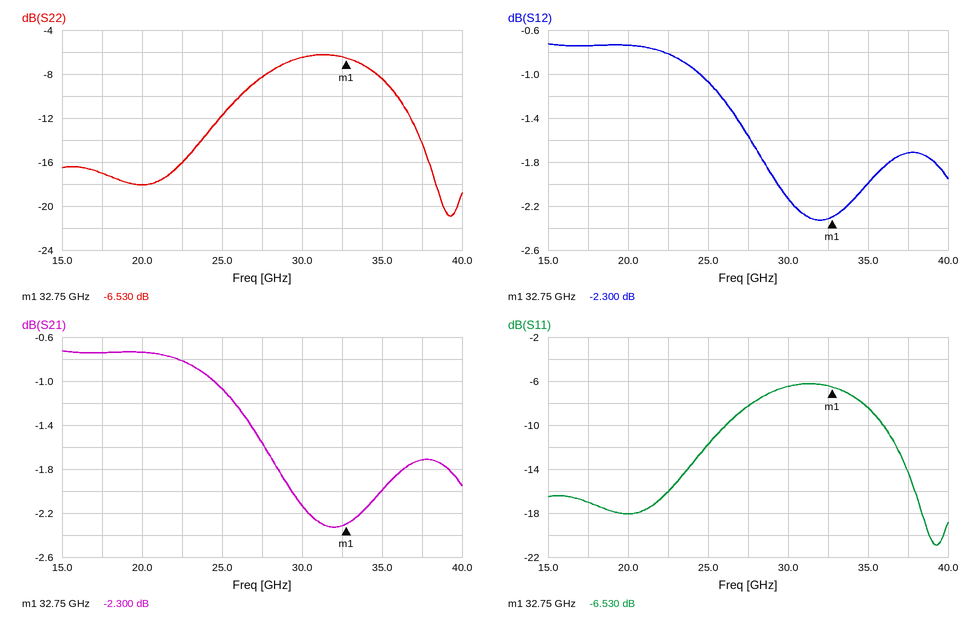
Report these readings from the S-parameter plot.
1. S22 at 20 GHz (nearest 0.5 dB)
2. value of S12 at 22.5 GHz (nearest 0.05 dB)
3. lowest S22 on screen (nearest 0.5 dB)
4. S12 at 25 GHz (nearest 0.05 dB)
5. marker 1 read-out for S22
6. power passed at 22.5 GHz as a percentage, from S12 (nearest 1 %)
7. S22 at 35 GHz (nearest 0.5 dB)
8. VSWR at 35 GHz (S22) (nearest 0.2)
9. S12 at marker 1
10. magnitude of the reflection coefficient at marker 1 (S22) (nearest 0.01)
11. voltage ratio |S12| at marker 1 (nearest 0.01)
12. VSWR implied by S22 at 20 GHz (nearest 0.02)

-18.0 dB
-0.80 dB
-21.0 dB
-1.05 dB
-6.530 dB
83 %
-8.5 dB
2.2
-2.300 dB
0.47
0.77
1.28
